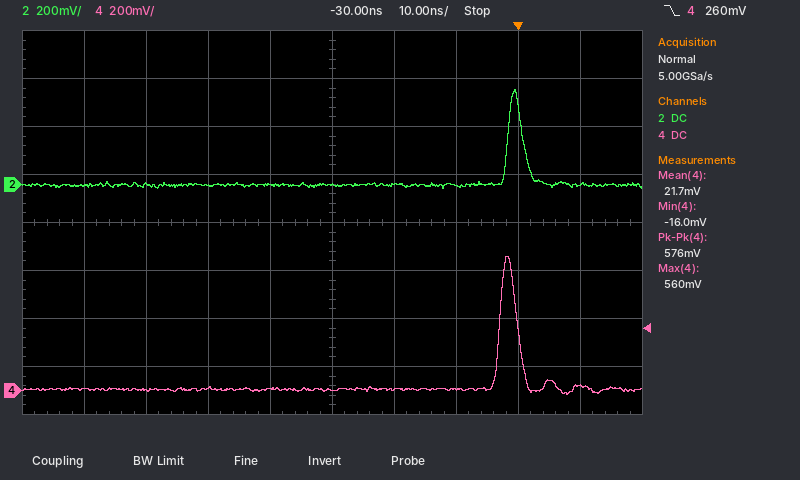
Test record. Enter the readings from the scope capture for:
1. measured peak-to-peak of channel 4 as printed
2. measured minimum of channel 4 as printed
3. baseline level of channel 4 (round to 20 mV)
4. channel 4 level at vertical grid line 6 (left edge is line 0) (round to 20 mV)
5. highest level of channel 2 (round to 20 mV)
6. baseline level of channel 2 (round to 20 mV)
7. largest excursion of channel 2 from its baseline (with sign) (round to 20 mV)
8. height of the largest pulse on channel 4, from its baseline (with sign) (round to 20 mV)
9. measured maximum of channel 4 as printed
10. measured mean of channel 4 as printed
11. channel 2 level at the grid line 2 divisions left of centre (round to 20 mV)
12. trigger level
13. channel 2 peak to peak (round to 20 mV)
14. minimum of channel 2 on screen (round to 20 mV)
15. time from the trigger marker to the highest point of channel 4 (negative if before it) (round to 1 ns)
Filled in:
576 mV
-16.0 mV
0 mV
0 mV
400 mV
0 mV
+400 mV
+560 mV
560 mV
21.7 mV
0 mV
260 mV
420 mV
-20 mV
-2 ns
